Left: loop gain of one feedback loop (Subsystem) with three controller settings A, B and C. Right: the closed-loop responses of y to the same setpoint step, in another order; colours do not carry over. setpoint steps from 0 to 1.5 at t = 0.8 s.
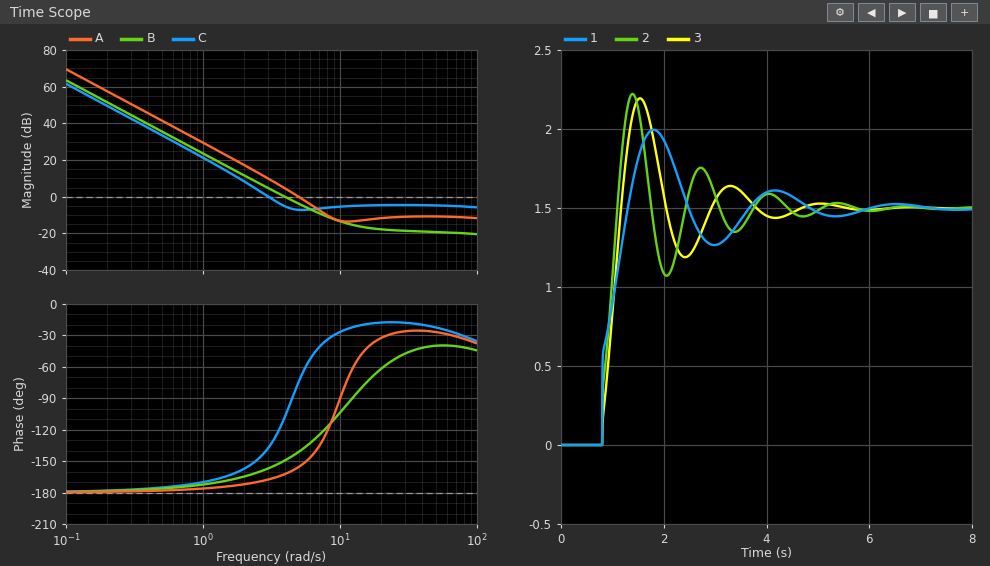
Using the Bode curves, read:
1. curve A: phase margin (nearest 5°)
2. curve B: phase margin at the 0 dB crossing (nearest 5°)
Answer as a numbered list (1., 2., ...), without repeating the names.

1. 25°
2. 30°
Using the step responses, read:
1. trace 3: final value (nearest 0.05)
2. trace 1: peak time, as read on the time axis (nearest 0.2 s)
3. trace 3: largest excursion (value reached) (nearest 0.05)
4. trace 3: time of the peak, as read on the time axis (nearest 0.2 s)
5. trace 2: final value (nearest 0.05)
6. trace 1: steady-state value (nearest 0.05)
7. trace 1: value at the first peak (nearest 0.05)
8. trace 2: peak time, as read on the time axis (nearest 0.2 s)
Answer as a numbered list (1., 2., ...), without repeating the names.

1. 1.50
2. 1.8 s
3. 2.20
4. 1.6 s
5. 1.50
6. 1.50
7. 2.00
8. 1.4 s
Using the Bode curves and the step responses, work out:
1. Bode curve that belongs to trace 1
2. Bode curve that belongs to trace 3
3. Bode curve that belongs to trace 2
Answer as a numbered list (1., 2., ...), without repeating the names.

1. C
2. B
3. A
